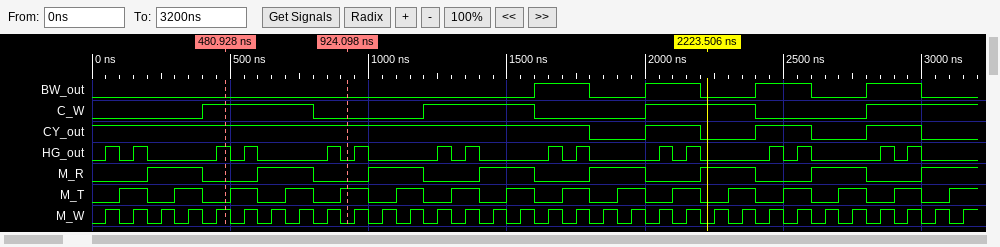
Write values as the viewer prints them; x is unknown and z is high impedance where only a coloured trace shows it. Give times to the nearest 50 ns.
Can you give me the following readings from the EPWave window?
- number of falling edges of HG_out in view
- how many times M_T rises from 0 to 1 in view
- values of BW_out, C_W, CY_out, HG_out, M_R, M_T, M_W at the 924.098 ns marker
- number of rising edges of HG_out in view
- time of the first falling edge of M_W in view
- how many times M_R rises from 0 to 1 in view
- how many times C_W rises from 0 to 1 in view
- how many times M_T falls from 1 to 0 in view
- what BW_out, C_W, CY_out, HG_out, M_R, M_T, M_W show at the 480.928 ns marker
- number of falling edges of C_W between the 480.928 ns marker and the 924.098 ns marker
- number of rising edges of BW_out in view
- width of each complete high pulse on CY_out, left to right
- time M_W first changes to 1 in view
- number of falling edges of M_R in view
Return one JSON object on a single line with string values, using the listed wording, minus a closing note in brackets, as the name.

{"number of falling edges of HG_out in view": "16", "how many times M_T rises from 0 to 1 in view": "16", "values of BW_out, C_W, CY_out, HG_out, M_R, M_T, M_W at the 924.098 ns marker": "BW_out=0, C_W=0, CY_out=1, HG_out=0, M_R=0, M_T=1, M_W=0", "number of rising edges of HG_out in view": "16", "time of the first falling edge of M_W in view": "100 ns", "how many times M_R rises from 0 to 1 in view": "8", "how many times C_W rises from 0 to 1 in view": "4", "how many times M_T falls from 1 to 0 in view": "15", "what BW_out, C_W, CY_out, HG_out, M_R, M_T, M_W show at the 480.928 ns marker": "BW_out=0, C_W=1, CY_out=1, HG_out=1, M_R=0, M_T=0, M_W=1", "number of falling edges of C_W between the 480.928 ns marker and the 924.098 ns marker": "1", "number of rising edges of BW_out in view": "4", "width of each complete high pulse on CY_out, left to right": "200 ns, 200 ns, 200 ns", "time M_W first changes to 1 in view": "50 ns", "number of falling edges of M_R in view": "7"}
